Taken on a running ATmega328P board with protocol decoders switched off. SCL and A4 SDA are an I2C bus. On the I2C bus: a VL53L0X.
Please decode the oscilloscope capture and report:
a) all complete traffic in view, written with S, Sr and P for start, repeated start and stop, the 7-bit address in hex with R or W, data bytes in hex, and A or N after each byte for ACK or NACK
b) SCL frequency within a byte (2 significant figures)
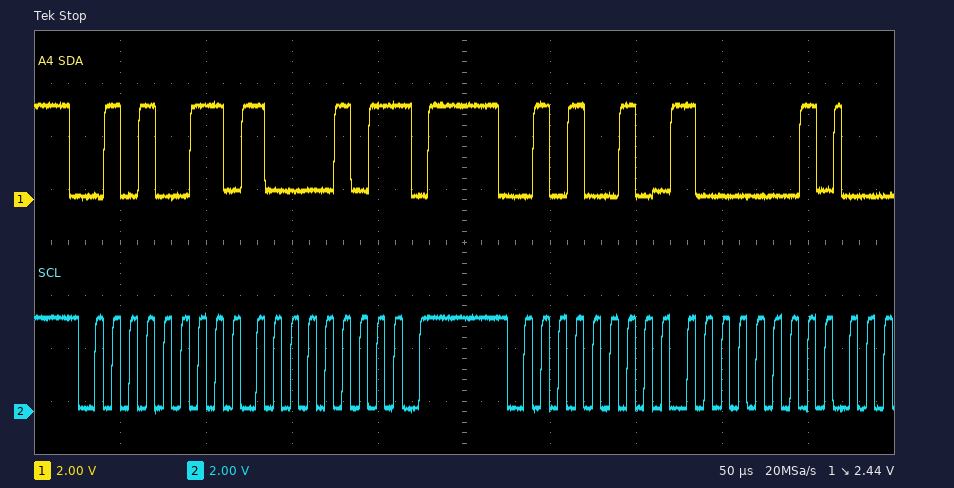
S 29R A 85 N P S 29W A 81 A
100 kHz
